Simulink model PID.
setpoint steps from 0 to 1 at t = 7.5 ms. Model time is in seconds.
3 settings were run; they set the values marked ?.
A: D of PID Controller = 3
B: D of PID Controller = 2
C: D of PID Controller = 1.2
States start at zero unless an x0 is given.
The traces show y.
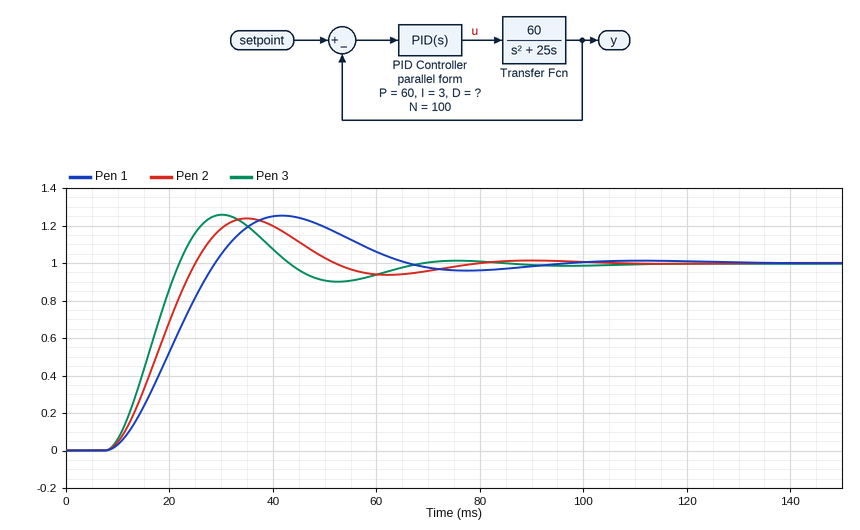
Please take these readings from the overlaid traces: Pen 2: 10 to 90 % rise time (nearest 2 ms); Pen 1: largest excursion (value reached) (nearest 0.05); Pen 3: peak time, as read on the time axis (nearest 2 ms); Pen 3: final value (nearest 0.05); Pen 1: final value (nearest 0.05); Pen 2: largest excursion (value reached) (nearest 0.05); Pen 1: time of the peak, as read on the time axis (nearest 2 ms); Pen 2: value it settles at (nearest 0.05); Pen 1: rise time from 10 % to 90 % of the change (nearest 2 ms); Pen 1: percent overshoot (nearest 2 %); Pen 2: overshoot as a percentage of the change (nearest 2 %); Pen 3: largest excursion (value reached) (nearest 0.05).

12 ms
1.25
30 ms
1.00
1.00
1.25
42 ms
1.00
14 ms
26 %
24 %
1.25
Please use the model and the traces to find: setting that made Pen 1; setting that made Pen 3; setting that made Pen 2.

C
A
B
